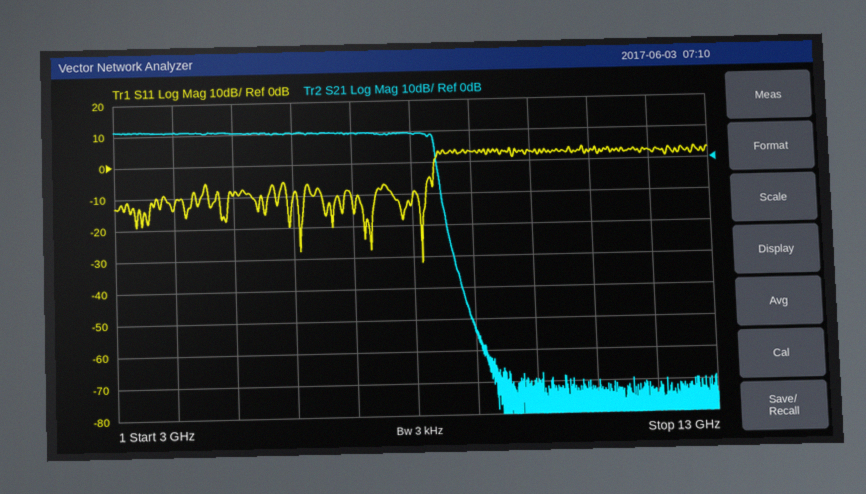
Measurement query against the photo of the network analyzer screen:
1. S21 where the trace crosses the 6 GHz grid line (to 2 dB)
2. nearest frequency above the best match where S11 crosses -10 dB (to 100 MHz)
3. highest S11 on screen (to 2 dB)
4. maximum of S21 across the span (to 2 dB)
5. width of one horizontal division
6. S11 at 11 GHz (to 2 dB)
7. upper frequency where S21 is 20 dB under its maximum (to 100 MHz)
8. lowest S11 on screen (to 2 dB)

10 dB
8.2 GHz
4 dB
12 dB
1 GHz
2 dB
8.5 GHz
-32 dB
